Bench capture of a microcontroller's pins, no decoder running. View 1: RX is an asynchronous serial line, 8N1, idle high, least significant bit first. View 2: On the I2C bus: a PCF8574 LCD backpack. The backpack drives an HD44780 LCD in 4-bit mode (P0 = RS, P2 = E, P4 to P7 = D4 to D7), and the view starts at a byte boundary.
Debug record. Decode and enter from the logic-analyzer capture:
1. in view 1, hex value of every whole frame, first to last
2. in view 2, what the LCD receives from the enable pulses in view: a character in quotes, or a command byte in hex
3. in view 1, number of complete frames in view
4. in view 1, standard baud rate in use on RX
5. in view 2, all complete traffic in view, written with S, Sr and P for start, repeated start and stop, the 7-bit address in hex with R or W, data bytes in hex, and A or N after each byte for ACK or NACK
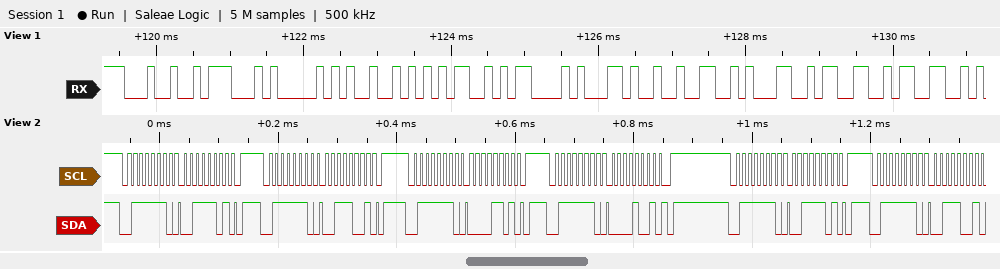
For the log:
24 47 50 52 4D 43 2C 32 31 33 33
'0'
11
9600 baud
S 3FW A 3D A P S 3FW A 39 A P S 3FW A 0D A P S 3FW A 09 A P S 3FW A 3D A P S 3FW A 39 A
